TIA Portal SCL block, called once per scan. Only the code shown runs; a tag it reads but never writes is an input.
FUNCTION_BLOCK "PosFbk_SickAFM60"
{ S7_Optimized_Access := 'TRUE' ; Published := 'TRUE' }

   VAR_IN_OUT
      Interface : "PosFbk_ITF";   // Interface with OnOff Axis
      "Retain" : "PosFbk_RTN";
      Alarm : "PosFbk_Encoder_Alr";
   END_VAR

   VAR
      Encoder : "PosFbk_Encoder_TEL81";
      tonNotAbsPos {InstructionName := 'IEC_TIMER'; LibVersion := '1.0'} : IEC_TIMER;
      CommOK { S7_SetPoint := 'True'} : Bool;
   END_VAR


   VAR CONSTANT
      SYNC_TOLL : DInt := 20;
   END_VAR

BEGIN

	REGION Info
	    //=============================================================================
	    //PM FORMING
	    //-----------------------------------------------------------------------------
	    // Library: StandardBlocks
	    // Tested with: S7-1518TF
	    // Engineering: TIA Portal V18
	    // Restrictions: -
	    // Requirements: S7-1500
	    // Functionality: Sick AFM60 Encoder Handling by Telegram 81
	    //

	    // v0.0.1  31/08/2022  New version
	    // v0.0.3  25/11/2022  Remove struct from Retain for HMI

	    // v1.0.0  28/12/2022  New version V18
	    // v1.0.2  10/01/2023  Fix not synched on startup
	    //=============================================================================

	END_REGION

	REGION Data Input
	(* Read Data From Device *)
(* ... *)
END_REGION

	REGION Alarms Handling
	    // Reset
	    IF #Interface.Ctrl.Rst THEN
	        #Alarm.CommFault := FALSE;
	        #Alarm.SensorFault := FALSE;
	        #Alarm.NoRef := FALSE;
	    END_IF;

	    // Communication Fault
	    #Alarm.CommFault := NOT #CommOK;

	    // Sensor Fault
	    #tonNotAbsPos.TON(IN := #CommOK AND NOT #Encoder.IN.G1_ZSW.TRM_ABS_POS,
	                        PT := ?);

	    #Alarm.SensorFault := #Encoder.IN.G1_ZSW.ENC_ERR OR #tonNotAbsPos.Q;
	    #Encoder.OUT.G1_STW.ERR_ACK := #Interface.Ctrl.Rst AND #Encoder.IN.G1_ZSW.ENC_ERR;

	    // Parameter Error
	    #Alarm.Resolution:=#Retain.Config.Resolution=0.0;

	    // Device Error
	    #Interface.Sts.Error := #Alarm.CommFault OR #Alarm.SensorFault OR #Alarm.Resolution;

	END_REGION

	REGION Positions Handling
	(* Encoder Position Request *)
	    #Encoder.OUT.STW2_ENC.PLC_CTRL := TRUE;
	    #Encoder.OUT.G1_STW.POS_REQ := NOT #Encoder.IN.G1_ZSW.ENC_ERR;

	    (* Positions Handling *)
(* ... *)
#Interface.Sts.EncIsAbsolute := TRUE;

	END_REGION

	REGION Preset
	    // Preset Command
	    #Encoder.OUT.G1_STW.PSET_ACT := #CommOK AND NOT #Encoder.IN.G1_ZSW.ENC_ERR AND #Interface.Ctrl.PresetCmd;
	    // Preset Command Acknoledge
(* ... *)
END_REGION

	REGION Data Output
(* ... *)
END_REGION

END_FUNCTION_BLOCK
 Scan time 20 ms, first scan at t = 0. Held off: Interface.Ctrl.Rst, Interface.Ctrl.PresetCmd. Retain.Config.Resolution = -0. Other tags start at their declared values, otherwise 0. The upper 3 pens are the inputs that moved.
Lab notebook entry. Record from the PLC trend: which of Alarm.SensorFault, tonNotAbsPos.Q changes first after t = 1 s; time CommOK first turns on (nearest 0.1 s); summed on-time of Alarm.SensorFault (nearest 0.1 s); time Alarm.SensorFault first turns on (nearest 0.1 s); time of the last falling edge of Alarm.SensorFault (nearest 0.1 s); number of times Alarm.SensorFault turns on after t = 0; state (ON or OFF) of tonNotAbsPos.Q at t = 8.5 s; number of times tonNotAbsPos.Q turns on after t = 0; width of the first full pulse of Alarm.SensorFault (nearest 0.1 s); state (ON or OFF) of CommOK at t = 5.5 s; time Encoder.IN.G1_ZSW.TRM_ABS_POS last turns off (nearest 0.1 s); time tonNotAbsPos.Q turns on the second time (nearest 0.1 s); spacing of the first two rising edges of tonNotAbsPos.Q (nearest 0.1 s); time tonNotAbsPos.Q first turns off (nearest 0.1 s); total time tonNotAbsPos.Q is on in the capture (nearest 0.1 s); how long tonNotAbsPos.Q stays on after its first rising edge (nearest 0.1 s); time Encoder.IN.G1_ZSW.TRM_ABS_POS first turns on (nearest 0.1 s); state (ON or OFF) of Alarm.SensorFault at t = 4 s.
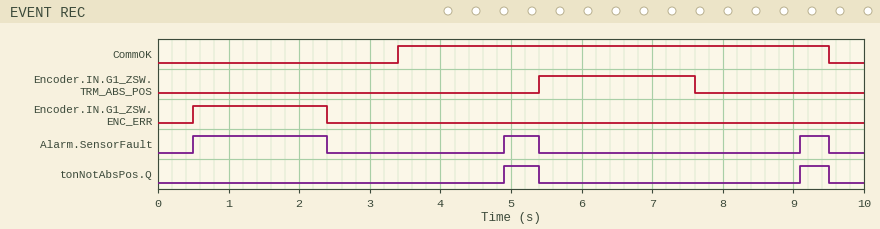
Alarm.SensorFault
3.4 s
2.8 s
0.5 s
9.5 s
3
OFF
2
1.9 s
ON
7.6 s
9.1 s
4.2 s
5.4 s
0.9 s
0.5 s
5.4 s
OFF
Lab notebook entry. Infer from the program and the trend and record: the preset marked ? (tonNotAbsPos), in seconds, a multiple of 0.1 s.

1.5 s
